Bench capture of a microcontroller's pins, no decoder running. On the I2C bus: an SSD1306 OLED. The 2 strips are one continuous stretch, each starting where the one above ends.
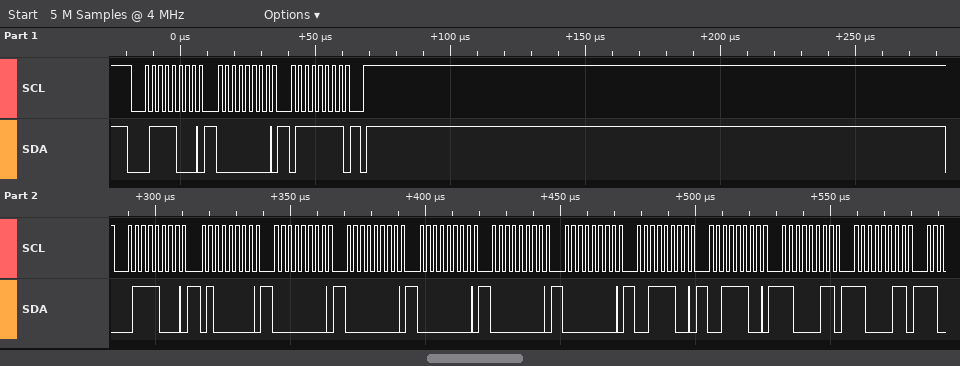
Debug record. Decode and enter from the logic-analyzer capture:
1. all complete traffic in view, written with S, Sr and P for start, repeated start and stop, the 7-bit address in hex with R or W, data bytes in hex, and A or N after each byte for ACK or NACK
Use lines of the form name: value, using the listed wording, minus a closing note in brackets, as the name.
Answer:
all complete traffic in view, written with S, Sr and P for start, repeated start and stop, the 7-bit address in hex with R or W, data bytes in hex, and A or N after each byte for ACK or NACK: S 3CW A 00 A 7F A P S 3CW A 40 A 00 A 00 A 00 A 00 A 00 A 3C A 3C A C3 A C3 A
